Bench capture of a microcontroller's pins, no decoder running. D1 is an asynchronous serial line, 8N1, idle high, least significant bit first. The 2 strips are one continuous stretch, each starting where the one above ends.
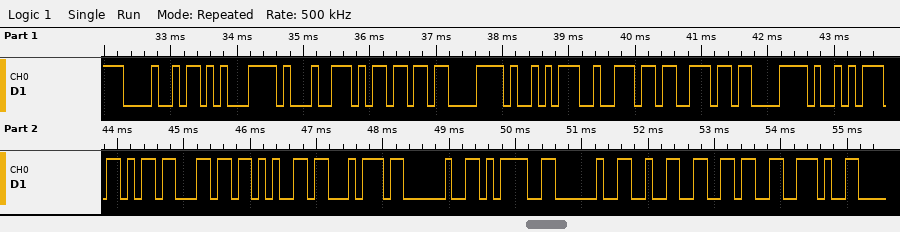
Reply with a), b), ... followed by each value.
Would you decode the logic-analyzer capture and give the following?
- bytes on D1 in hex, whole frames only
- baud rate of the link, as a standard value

a) 0x48 0xC5 0x91 0x6D 0xC3 0xA9 0x72 0x73 0xC3 0xA9 0x6B 0x6C 0x65 0x74 0x20 0x3D 0x20 0x32 0x36 0x2E
b) 9600 baud
